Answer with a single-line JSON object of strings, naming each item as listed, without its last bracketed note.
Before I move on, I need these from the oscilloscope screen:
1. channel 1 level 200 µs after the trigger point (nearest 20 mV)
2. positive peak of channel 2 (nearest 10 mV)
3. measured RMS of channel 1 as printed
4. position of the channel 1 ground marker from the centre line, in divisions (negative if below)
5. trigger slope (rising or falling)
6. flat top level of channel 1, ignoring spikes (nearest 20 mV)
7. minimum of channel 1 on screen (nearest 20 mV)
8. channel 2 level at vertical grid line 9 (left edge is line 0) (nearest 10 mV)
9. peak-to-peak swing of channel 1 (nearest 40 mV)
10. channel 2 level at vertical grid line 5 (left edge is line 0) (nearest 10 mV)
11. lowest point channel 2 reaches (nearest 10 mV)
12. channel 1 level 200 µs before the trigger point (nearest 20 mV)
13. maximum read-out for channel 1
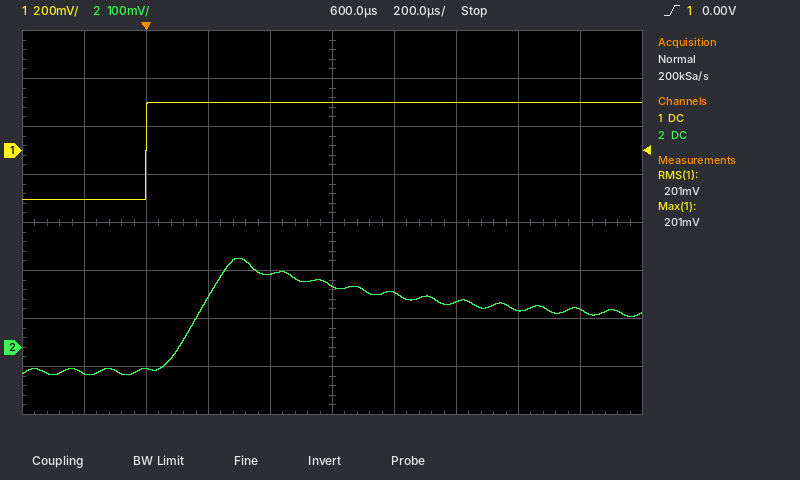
{"channel 1 level 200 µs after the trigger point": "200 mV", "positive peak of channel 2": "190 mV", "measured RMS of channel 1 as printed": "201 mV", "position of the channel 1 ground marker from the centre line, in divisions": "+1.5 div", "trigger slope": "rising", "flat top level of channel 1, ignoring spikes": "200 mV", "minimum of channel 1 on screen": "-200 mV", "channel 2 level at vertical grid line 9 (left edge is line 0)": "80 mV", "peak-to-peak swing of channel 1": "400 mV", "channel 2 level at vertical grid line 5 (left edge is line 0)": "130 mV", "lowest point channel 2 reaches": "-60 mV", "channel 1 level 200 µs before the trigger point": "-200 mV", "maximum read-out for channel 1": "201 mV"}
